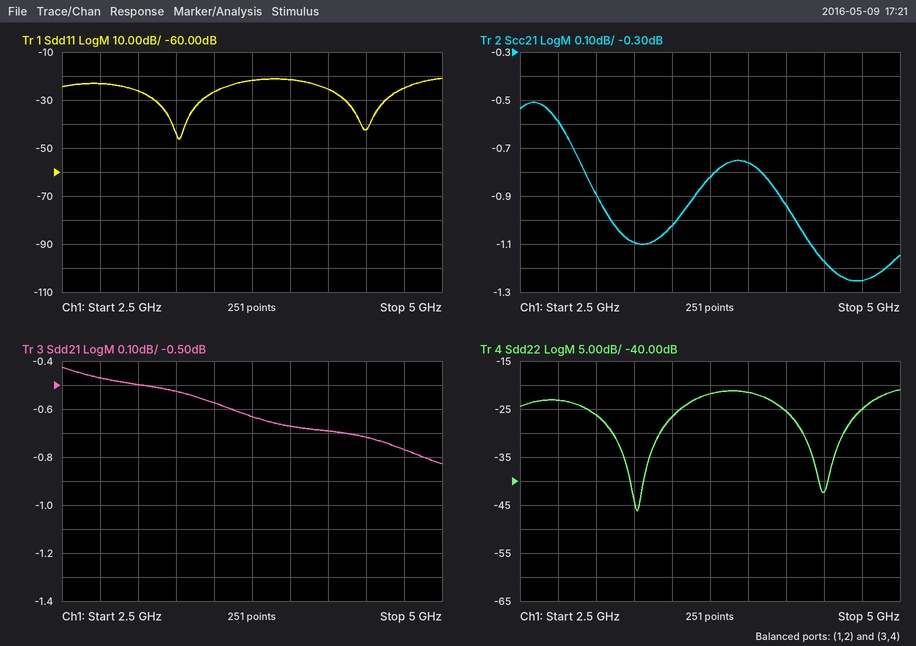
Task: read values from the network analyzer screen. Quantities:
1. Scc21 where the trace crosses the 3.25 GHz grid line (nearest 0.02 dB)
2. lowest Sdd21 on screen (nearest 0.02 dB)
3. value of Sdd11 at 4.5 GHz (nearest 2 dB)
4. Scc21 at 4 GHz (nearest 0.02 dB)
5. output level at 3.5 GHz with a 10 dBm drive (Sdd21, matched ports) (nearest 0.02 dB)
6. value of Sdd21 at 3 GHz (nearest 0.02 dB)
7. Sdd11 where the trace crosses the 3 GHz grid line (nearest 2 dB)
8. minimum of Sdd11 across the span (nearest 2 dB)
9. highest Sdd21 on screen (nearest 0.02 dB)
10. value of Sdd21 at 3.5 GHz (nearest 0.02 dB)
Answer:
-1.10 dB
-0.82 dB
-42 dB
-0.76 dB
9.42 dBm
-0.50 dB
-26 dB
-46 dB
-0.42 dB
-0.58 dB
